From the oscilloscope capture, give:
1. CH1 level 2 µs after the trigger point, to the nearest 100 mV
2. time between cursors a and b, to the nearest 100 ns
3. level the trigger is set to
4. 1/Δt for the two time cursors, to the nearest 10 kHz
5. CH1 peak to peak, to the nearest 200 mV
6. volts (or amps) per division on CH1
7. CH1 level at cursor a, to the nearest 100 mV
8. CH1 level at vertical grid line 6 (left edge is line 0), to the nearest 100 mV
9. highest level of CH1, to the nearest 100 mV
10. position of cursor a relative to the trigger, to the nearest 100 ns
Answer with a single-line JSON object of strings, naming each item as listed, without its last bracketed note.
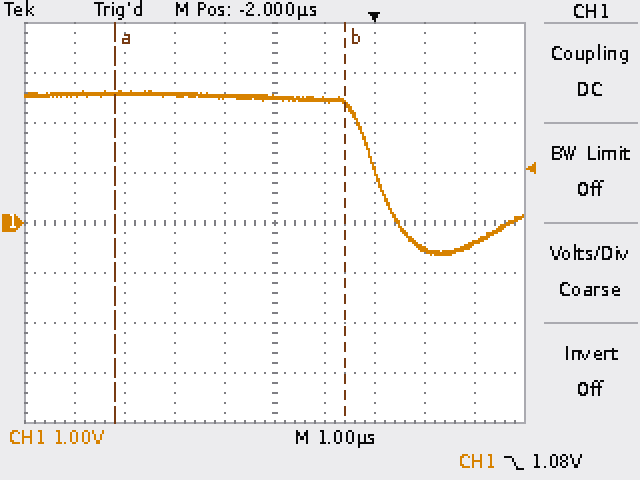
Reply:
{"CH1 level 2 µs after the trigger point, to the nearest 100 mV": "-400 mV", "time between cursors a and b, to the nearest 100 ns": "4.6 µs", "level the trigger is set to": "1.08 V", "1/Δt for the two time cursors, to the nearest 10 kHz": "220 kHz", "CH1 peak to peak, to the nearest 200 mV": "3.2 V", "volts (or amps) per division on CH1": "1 V", "CH1 level at cursor a, to the nearest 100 mV": "2.6 V", "CH1 level at vertical grid line 6 (left edge is line 0), to the nearest 100 mV": "2.5 V", "highest level of CH1, to the nearest 100 mV": "2.6 V", "position of cursor a relative to the trigger, to the nearest 100 ns": "-5.2 µs"}
